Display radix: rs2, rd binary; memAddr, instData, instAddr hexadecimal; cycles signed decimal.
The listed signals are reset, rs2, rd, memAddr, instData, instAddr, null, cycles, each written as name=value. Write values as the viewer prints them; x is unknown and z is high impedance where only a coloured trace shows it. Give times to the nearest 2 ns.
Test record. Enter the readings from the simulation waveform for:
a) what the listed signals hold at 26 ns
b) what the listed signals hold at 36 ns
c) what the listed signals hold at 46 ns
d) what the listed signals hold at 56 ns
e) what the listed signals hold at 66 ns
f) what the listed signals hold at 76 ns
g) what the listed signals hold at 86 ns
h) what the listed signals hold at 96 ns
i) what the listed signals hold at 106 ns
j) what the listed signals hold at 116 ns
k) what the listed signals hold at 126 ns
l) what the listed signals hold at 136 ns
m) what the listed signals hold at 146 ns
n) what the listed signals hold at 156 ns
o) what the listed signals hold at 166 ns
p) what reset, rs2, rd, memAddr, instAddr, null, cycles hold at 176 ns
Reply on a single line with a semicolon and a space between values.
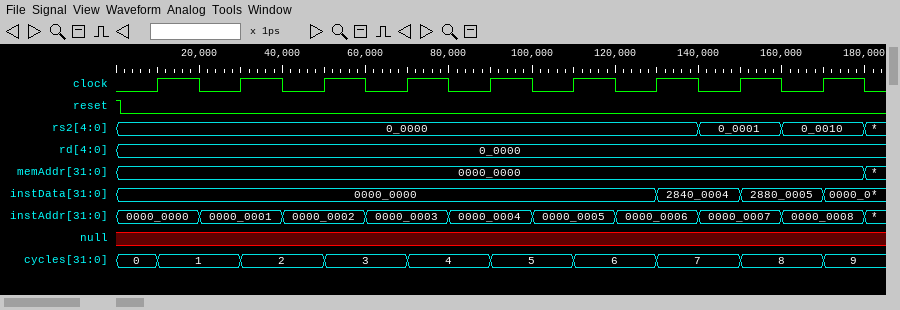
reset=0, rs2=0_0000, rd=0_0000, memAddr=0000_0000, instData=0000_0000, instAddr=0000_0001, null=x, cycles=1; reset=0, rs2=0_0000, rd=0_0000, memAddr=0000_0000, instData=0000_0000, instAddr=0000_0001, null=x, cycles=2; reset=0, rs2=0_0000, rd=0_0000, memAddr=0000_0000, instData=0000_0000, instAddr=0000_0002, null=x, cycles=2; reset=0, rs2=0_0000, rd=0_0000, memAddr=0000_0000, instData=0000_0000, instAddr=0000_0002, null=x, cycles=3; reset=0, rs2=0_0000, rd=0_0000, memAddr=0000_0000, instData=0000_0000, instAddr=0000_0003, null=x, cycles=3; reset=0, rs2=0_0000, rd=0_0000, memAddr=0000_0000, instData=0000_0000, instAddr=0000_0003, null=x, cycles=4; reset=0, rs2=0_0000, rd=0_0000, memAddr=0000_0000, instData=0000_0000, instAddr=0000_0004, null=x, cycles=4; reset=0, rs2=0_0000, rd=0_0000, memAddr=0000_0000, instData=0000_0000, instAddr=0000_0004, null=x, cycles=5; reset=0, rs2=0_0000, rd=0_0000, memAddr=0000_0000, instData=0000_0000, instAddr=0000_0005, null=x, cycles=5; reset=0, rs2=0_0000, rd=0_0000, memAddr=0000_0000, instData=0000_0000, instAddr=0000_0005, null=x, cycles=6; reset=0, rs2=0_0000, rd=0_0000, memAddr=0000_0000, instData=0000_0000, instAddr=0000_0006, null=x, cycles=6; reset=0, rs2=0_0000, rd=0_0000, memAddr=0000_0000, instData=2840_0004, instAddr=0000_0006, null=x, cycles=7; reset=0, rs2=0_0001, rd=0_0000, memAddr=0000_0000, instData=2840_0004, instAddr=0000_0007, null=x, cycles=7; reset=0, rs2=0_0001, rd=0_0000, memAddr=0000_0000, instData=2880_0005, instAddr=0000_0007, null=x, cycles=8; reset=0, rs2=0_0010, rd=0_0000, memAddr=0000_0000, instData=2880_0005, instAddr=0000_0008, null=x, cycles=8; reset=0, rs2=0_0010, rd=0_0000, memAddr=0000_0000, instAddr=0000_0008, null=x, cycles=9
